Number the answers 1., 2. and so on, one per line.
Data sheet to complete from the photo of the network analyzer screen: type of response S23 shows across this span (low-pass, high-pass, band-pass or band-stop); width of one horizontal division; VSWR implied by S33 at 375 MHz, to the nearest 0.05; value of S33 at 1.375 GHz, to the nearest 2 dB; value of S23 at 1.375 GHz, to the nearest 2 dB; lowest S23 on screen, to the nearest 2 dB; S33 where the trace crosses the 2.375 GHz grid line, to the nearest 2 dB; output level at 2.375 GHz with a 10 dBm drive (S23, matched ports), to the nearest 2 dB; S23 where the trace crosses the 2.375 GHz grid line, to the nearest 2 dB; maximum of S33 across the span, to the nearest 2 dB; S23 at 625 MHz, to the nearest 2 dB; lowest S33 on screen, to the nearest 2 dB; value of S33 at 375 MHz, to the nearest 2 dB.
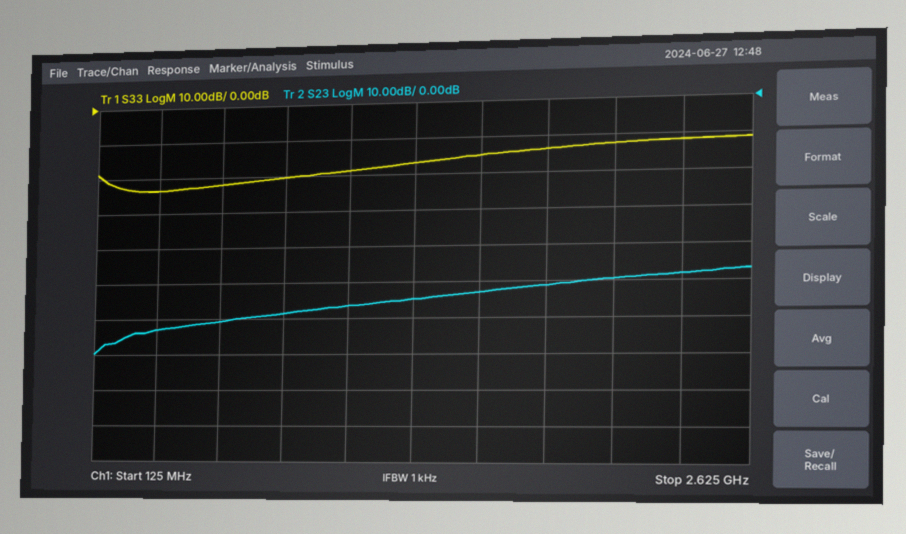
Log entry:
1. high-pass
2. 250 MHz
3. 1.15
4. -16 dB
5. -54 dB
6. -70 dB
7. -12 dB
8. -38 dBm
9. -48 dB
10. -12 dB
11. -60 dB
12. -24 dB
13. -24 dB
